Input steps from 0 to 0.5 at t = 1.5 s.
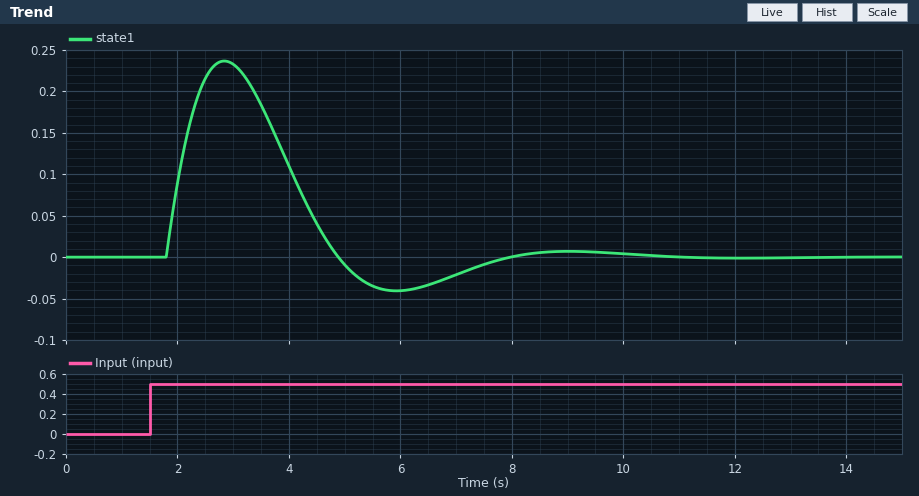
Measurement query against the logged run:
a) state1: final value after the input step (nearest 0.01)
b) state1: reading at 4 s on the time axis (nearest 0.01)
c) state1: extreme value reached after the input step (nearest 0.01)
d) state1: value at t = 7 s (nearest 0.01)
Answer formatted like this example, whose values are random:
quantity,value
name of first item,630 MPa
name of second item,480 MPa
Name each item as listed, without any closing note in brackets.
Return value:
quantity,value
state1: final value after the input step,0.00
state1: reading at 4 s on the time axis,0.11
state1: extreme value reached after the input step,0.24
state1: value at t = 7 s,-0.02
